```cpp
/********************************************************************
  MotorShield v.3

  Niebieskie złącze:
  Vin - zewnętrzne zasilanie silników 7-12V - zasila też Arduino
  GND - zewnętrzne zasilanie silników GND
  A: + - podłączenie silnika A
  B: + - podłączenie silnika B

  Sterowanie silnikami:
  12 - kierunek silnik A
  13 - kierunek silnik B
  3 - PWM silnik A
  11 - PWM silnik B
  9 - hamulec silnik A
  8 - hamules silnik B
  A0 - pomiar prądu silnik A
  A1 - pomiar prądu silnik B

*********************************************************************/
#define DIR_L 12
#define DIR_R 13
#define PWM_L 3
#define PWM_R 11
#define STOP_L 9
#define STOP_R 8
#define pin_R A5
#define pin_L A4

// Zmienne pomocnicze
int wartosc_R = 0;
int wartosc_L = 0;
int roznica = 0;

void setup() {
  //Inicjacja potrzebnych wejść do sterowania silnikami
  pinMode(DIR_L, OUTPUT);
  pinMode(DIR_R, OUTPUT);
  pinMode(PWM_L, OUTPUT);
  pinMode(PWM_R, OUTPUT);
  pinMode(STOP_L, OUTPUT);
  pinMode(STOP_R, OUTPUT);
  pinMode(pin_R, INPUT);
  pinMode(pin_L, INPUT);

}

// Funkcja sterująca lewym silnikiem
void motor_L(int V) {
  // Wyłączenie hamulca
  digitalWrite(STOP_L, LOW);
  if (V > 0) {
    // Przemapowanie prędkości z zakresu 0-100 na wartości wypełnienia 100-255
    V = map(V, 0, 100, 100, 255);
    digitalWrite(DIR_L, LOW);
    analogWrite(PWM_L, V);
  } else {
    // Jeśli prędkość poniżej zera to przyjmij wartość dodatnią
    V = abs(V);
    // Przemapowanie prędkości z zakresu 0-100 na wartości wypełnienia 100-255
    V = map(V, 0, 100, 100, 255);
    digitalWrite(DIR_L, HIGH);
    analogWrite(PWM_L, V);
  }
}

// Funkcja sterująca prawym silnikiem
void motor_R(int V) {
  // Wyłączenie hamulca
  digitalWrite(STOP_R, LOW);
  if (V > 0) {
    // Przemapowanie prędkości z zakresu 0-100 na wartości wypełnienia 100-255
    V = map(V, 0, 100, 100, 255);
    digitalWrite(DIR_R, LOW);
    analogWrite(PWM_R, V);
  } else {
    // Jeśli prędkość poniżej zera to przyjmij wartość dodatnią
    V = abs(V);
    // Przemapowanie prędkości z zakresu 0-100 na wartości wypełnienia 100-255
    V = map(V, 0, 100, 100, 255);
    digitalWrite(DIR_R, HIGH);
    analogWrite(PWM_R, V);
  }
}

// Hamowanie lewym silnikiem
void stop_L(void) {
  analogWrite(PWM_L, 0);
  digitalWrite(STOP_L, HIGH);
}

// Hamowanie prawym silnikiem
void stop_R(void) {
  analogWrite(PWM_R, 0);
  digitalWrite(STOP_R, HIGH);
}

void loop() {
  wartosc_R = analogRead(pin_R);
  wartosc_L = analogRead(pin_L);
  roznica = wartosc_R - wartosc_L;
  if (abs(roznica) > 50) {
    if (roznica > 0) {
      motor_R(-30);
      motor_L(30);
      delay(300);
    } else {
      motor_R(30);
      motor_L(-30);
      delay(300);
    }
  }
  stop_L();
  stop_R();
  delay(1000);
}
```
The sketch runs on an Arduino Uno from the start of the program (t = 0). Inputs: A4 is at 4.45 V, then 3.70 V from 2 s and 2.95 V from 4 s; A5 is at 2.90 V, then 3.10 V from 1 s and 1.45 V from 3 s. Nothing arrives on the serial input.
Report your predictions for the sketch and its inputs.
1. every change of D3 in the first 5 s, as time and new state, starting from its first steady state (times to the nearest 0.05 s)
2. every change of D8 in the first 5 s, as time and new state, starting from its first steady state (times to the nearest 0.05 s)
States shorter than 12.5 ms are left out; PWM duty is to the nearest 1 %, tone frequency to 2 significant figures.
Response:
0 s PWM 57 %; 0.3 s low; 1.3 s PWM 57 %; 1.6 s low; 2.6 s PWM 57 %; 2.9 s low; 3.9 s PWM 57 %; 4.2 s low
0 s low; 0.3 s high; 1.3 s low; 1.6 s high; 2.6 s low; 2.9 s high; 3.9 s low; 4.2 s high
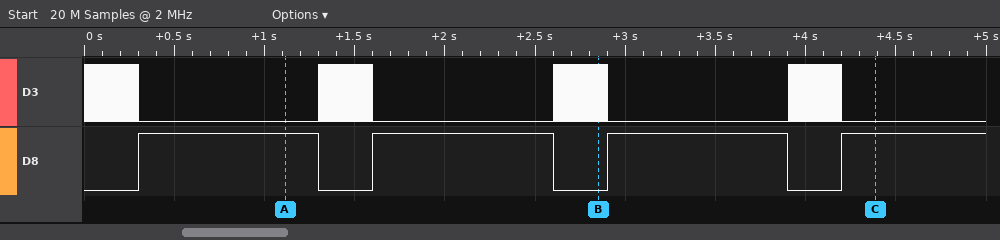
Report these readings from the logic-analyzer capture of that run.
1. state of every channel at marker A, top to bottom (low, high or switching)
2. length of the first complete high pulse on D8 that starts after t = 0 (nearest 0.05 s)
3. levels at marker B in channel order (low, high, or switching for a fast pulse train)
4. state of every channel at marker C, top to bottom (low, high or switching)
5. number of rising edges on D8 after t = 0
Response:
D3 low, D8 high
1.00 s
D3 switching, D8 low
D3 low, D8 high
4
